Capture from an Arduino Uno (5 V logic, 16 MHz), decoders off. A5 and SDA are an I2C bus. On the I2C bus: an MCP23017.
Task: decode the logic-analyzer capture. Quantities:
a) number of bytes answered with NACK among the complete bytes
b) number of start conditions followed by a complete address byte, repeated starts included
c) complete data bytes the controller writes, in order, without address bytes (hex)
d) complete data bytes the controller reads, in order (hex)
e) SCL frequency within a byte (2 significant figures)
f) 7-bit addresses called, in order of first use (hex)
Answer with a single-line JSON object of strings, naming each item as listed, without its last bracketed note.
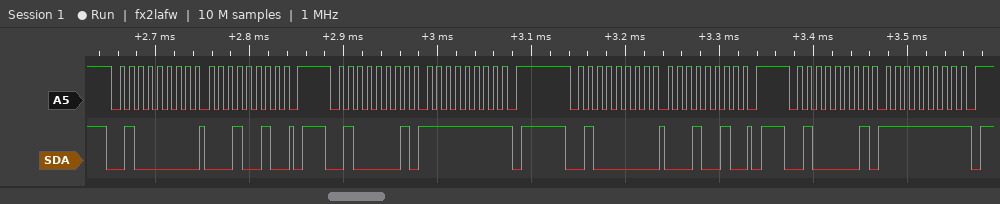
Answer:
{"number of bytes answered with NACK among the complete bytes": "2", "number of start conditions followed by a complete address byte, repeated starts included": "4", "complete data bytes the controller writes, in order, without address bytes": "12 12", "complete data bytes the controller reads, in order": "FF FF", "SCL frequency within a byte": "100 kHz", "7-bit addresses called, in order of first use": "0x20"}
